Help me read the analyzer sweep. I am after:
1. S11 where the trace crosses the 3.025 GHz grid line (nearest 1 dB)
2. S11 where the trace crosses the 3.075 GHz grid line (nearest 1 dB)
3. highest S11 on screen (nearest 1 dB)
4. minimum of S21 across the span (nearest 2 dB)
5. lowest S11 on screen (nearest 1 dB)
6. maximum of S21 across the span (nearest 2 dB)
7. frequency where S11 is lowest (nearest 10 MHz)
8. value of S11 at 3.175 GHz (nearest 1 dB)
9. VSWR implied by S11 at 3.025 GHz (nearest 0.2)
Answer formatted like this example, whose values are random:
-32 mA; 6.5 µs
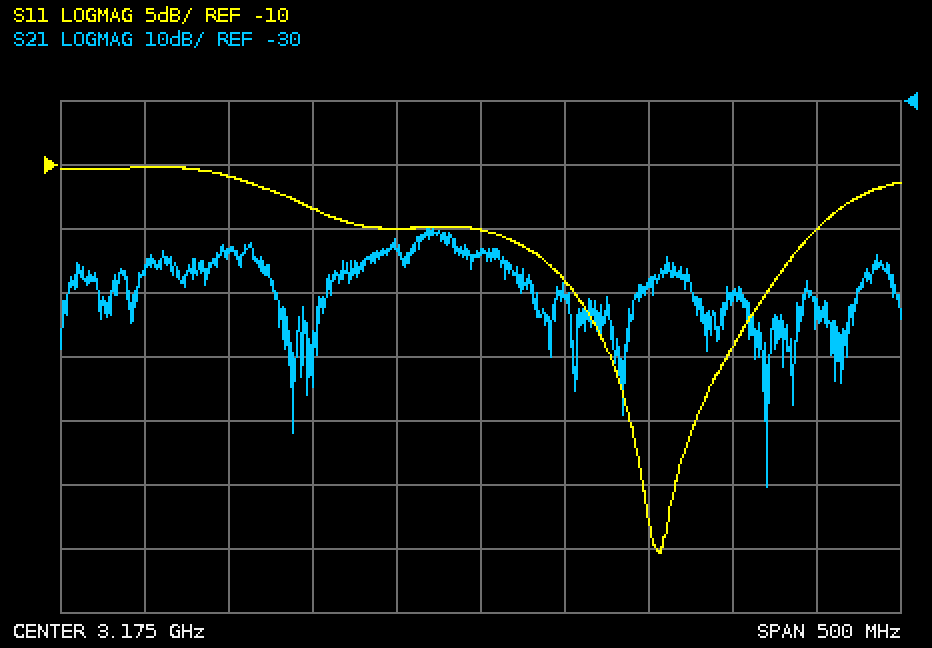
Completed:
-11 dB; -13 dB; -10 dB; -90 dB; -40 dB; -50 dB; 3.28 GHz; -15 dB; 1.8
